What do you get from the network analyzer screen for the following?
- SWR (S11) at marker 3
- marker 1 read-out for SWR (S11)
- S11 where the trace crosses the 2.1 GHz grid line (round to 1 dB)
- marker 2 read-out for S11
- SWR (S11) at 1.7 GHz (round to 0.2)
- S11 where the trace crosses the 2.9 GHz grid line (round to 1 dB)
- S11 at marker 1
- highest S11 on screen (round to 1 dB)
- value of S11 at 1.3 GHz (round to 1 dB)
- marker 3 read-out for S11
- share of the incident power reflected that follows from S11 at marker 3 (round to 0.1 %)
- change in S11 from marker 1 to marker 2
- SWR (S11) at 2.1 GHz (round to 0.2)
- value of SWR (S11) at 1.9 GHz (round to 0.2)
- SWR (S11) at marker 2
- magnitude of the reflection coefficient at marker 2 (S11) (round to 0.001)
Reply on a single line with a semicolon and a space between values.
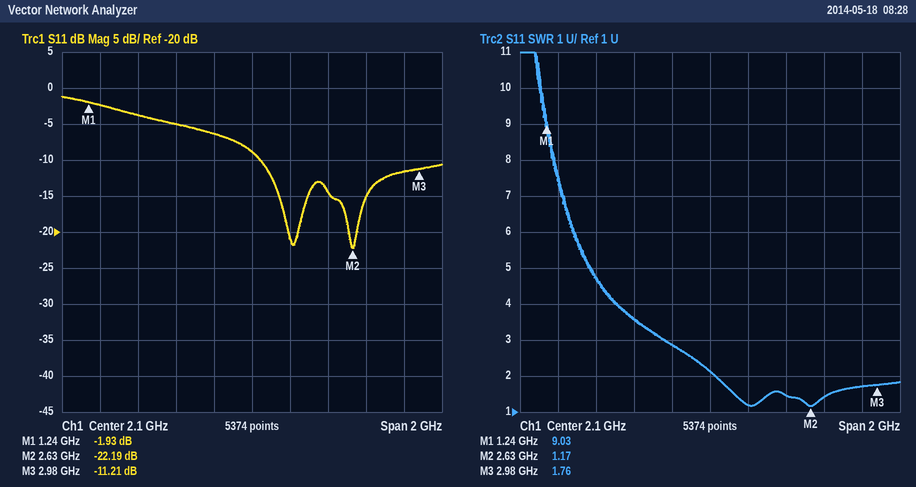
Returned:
1.76; 9.03; -9 dB; -22.19 dB; 3.6; -12 dB; -1.93 dB; -1 dB; -2 dB; -11.21 dB; 7.6 %; -20.26 dB; 2.2; 2.8; 1.17; 0.078
